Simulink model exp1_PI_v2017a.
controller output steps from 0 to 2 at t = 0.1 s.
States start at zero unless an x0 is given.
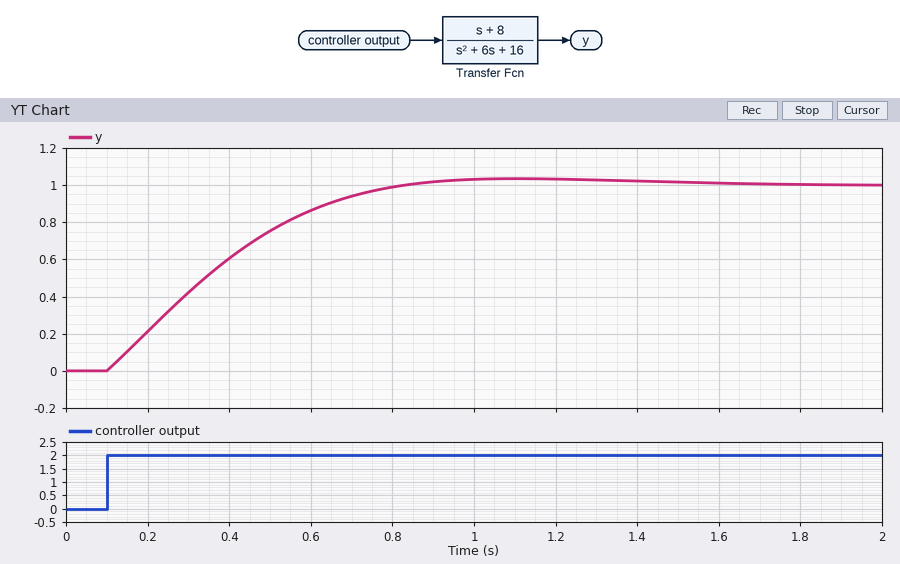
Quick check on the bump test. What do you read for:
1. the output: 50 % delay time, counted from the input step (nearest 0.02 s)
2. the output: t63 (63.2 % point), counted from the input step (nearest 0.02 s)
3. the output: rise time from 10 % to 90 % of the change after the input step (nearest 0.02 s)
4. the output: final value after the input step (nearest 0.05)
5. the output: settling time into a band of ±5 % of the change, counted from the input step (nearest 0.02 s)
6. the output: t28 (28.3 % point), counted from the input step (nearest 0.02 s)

0.24 s
0.32 s
0.50 s
1.00
0.62 s
0.14 s
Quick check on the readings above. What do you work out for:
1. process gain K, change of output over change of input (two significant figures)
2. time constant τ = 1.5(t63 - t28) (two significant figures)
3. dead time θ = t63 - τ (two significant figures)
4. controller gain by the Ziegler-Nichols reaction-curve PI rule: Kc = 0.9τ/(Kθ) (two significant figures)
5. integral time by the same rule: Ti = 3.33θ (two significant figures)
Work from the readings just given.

0.50
0.27 s
0.050 s
9.7
0.17 s
